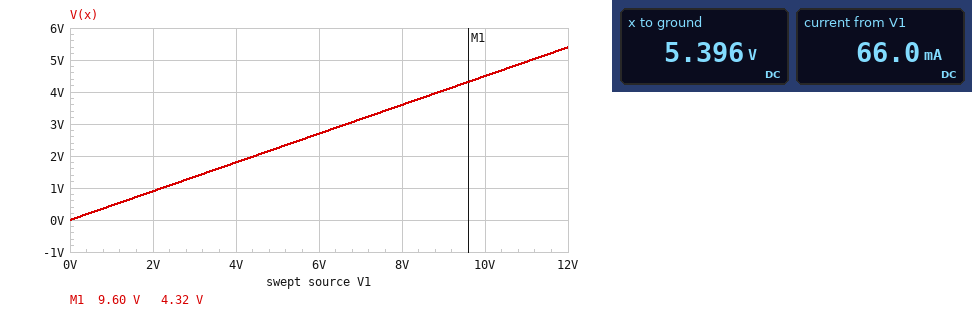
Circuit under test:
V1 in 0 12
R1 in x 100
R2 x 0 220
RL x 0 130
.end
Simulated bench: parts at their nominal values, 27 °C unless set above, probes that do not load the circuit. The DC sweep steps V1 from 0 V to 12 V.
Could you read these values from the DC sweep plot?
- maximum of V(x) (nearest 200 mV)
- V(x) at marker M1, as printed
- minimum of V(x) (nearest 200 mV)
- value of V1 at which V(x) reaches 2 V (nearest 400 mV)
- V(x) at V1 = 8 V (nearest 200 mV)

5.4 V
4.32 V
0 V
4.4 V
3.6 V
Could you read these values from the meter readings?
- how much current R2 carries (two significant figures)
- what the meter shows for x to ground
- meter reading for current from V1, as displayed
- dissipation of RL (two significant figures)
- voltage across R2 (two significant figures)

25 mA
5.396 V
66.0 mA
220 mW
5.4 V
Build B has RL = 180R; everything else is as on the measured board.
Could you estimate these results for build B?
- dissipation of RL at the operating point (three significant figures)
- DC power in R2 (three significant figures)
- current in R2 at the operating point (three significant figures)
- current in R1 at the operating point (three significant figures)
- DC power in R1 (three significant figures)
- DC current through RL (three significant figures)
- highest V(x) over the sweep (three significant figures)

198 mW
162 mW
27.1 mA
60.3 mA
364 mW
33.2 mA
5.97 V
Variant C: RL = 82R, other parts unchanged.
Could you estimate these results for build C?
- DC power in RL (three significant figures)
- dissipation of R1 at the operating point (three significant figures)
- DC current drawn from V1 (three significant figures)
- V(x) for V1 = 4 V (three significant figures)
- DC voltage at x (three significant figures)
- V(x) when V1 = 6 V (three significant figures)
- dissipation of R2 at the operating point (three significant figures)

246 mW
564 mW
75.1 mA
1.50 V
4.49 V
2.24 V
91.5 mW
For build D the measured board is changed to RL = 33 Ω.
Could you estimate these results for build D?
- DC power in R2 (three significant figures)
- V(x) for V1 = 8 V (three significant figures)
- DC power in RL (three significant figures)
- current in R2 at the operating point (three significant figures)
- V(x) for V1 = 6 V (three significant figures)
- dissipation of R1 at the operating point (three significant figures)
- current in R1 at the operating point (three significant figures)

32.5 mW
1.78 V
217 mW
12.2 mA
1.34 V
869 mW
93.2 mA
